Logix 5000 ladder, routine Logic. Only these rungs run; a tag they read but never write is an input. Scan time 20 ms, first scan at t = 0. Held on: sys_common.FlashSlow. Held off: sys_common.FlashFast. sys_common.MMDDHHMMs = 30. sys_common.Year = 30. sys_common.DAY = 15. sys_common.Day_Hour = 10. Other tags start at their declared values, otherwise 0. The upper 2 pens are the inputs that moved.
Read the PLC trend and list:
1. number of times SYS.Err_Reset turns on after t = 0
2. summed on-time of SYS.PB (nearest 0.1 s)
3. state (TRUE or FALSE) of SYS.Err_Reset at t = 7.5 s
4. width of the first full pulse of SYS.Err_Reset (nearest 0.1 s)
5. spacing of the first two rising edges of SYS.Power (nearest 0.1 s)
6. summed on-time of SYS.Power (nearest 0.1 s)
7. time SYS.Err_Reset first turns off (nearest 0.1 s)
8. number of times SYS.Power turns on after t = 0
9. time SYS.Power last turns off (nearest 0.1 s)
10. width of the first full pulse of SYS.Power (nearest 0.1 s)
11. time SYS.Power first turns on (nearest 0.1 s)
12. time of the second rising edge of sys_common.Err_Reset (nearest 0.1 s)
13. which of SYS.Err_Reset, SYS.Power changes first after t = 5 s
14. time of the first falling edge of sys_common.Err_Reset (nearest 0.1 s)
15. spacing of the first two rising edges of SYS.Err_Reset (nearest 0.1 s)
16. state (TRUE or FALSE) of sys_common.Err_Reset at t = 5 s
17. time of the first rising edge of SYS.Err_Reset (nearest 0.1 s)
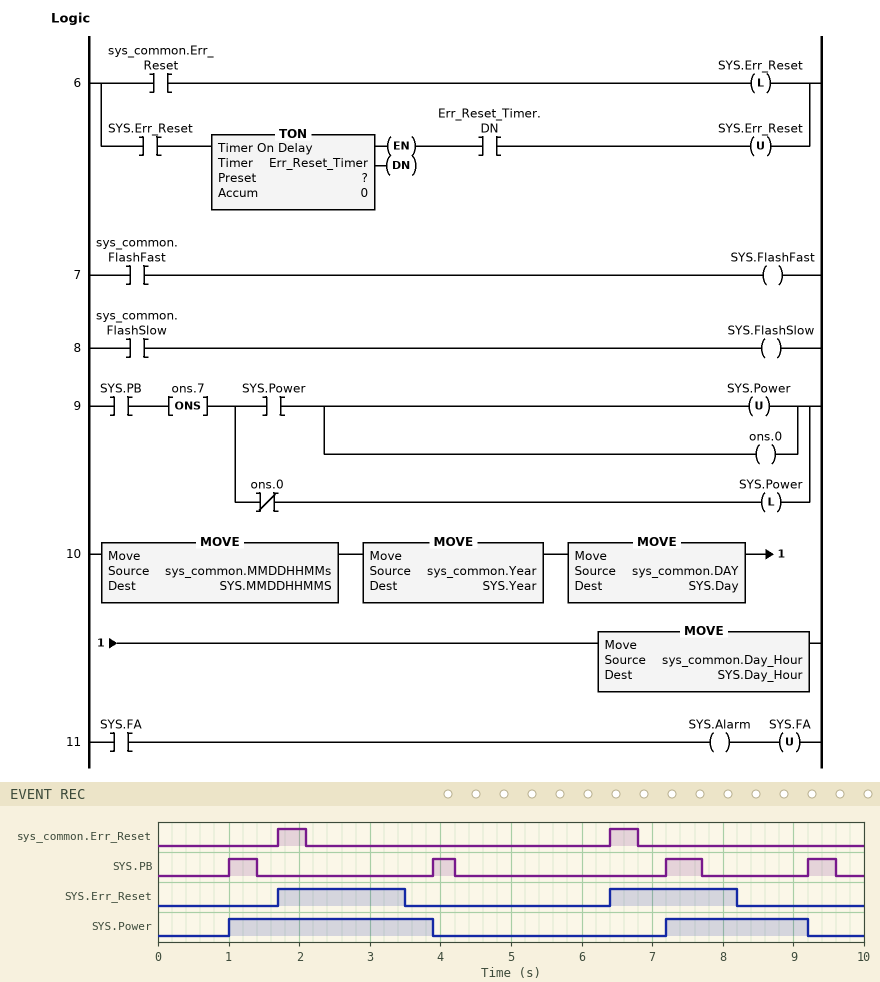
2
1.6 s
TRUE
1.8 s
6.2 s
4.9 s
3.5 s
2
9.2 s
2.9 s
1.0 s
6.4 s
SYS.Err_Reset
2.1 s
4.7 s
FALSE
1.7 s
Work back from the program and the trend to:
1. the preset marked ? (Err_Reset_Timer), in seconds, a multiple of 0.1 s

1.8 s
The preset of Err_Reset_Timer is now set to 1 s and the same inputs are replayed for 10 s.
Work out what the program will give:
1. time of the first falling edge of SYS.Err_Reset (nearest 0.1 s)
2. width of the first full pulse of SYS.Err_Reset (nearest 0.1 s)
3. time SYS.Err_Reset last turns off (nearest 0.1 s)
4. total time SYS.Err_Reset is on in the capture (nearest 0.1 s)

2.7 s
1.0 s
7.4 s
2.0 s
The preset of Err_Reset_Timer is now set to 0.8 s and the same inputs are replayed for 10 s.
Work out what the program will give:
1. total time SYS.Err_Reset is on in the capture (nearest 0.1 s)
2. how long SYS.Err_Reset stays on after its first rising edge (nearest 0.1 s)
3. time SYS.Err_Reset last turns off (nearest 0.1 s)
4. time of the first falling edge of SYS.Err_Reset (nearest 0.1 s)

1.6 s
0.8 s
7.2 s
2.5 s
